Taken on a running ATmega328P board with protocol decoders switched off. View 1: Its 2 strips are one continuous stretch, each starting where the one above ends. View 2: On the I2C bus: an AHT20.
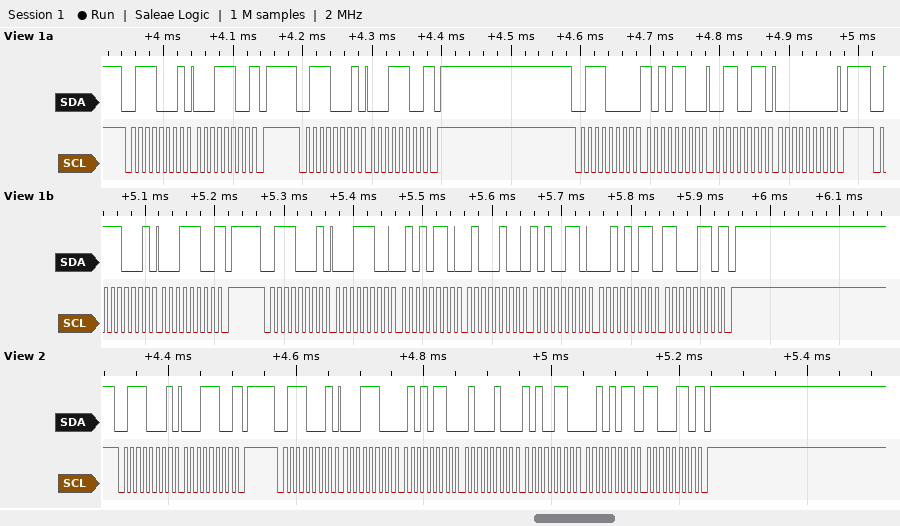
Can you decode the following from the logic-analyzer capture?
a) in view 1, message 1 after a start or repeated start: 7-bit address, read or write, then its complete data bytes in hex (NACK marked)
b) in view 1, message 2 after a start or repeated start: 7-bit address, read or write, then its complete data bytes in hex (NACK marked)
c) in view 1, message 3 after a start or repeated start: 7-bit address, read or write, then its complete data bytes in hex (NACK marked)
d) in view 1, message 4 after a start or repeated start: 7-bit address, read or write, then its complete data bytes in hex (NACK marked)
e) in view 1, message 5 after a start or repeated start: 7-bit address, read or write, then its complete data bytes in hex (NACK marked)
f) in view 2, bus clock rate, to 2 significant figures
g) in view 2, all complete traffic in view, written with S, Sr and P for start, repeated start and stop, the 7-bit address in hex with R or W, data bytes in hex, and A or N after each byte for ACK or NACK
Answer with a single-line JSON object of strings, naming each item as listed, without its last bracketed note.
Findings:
{"in view 1, message 1 after a start or repeated start: 7-bit address, read or write, then its complete data bytes in hex": "0x38 read: 1C NACK", "in view 1, message 2 after a start or repeated start: 7-bit address, read or write, then its complete data bytes in hex": "0x38 read: 1C NACK", "in view 1, message 3 after a start or repeated start: 7-bit address, read or write, then its complete data bytes in hex": "0x38 write: AC 33 00", "in view 1, message 4 after a start or repeated start: 7-bit address, read or write, then its complete data bytes in hex": "0x38 read: 1C NACK", "in view 1, message 5 after a start or repeated start: 7-bit address, read or write, then its complete data bytes in hex": "0x38 read: 1C 56 44 A6 2B C6 NACK", "in view 2, bus clock rate, to 2 significant figures": "100 kHz", "in view 2, all complete traffic in view, written with S, Sr and P for start, repeated start and stop, the 7-bit address in hex with R or W, data bytes in hex, and A or N after each byte for ACK or NACK": "S 38R A 1C N P S 38R A 1C A 56 A 44 A A6 A 2B A C6 N P"}
